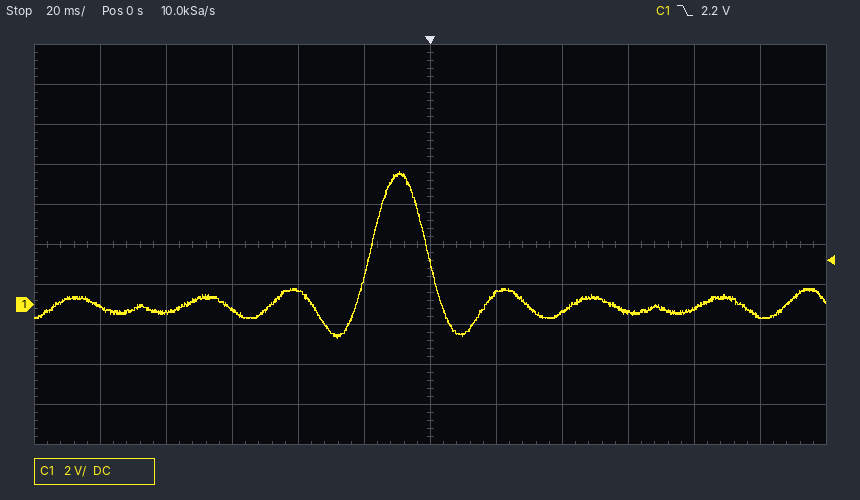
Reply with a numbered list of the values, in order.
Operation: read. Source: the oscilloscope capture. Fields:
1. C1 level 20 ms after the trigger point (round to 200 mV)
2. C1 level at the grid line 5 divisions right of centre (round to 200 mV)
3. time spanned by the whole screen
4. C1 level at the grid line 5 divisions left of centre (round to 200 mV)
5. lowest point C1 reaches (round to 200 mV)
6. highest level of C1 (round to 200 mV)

1. 600 mV
2. -600 mV
3. 240 ms
4. -200 mV
5. -1.6 V
6. 6.6 V
